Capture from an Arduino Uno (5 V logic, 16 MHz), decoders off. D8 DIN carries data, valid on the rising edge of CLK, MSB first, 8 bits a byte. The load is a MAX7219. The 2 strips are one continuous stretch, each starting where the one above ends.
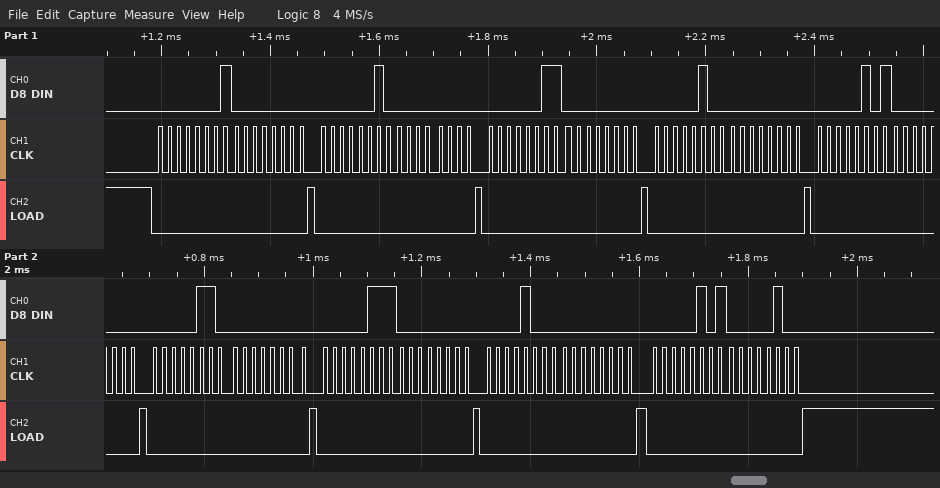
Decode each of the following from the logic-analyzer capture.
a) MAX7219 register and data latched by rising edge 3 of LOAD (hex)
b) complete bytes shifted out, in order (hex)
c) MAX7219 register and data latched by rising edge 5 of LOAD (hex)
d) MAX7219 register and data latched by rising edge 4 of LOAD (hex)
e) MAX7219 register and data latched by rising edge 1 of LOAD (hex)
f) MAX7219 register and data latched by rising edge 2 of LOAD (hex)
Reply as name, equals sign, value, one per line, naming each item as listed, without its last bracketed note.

MAX7219 register and data latched by rising edge 3 of LOAD = register 0x3, data 0x00
complete bytes shifted out, in order = 01 00 02 00 03 00 04 00 05 00 06 00 07 00 08 00 05 04
MAX7219 register and data latched by rising edge 5 of LOAD = register 0x5, data 0x00
MAX7219 register and data latched by rising edge 4 of LOAD = register 0x4, data 0x00
MAX7219 register and data latched by rising edge 1 of LOAD = register 0x1, data 0x00
MAX7219 register and data latched by rising edge 2 of LOAD = register 0x2, data 0x00
